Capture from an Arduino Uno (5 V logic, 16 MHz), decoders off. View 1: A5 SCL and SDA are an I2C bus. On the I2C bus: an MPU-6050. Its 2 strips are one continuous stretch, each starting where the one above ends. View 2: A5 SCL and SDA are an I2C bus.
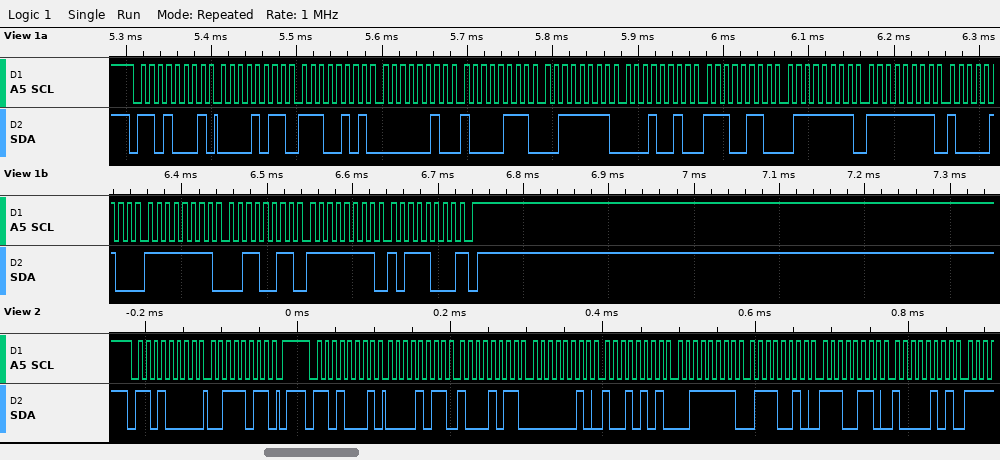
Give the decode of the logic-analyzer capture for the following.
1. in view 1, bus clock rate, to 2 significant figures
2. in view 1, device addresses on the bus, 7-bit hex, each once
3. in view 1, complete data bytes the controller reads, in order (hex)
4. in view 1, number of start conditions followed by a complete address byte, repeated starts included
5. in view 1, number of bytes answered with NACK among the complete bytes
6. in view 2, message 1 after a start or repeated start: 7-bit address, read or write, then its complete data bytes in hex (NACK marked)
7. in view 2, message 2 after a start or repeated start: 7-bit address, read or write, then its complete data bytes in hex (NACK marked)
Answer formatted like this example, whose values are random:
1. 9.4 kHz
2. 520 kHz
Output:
1. 100 kHz
2. 0x68
3. 0B E5 02 87 3F 12 E6 7F FF 84 FF 33 FF B8
4. 1
5. 1
6. 0x68 write: 3B
7. 0x68 read: 0B 8B 02 95 3F 72 E6 85
